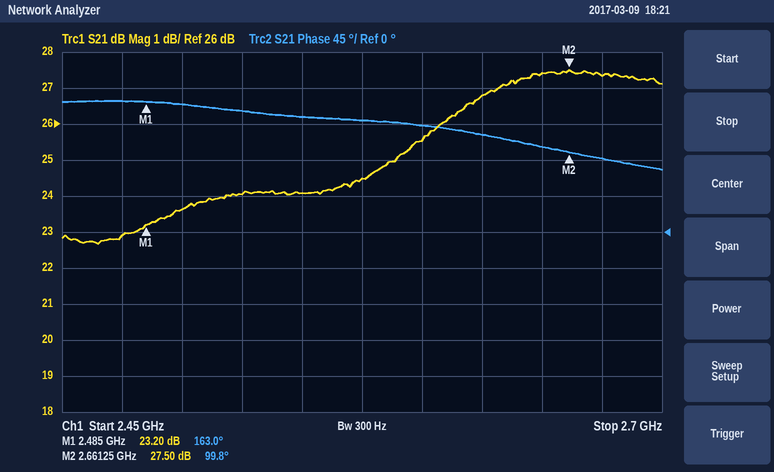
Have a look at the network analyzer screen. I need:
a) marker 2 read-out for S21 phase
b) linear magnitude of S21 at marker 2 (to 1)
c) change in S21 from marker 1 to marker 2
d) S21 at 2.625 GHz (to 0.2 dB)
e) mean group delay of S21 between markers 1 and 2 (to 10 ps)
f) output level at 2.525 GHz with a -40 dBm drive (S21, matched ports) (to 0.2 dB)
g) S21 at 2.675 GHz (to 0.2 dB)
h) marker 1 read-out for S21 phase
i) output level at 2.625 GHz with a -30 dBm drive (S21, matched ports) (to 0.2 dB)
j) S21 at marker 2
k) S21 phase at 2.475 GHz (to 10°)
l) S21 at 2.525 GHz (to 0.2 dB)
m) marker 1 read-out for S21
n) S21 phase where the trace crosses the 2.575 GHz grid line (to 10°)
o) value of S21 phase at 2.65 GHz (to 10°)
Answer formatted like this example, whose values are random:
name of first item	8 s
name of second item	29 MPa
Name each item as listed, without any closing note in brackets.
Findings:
marker 2 read-out for S21 phase	99.8°
linear magnitude of S21 at marker 2	24
change in S21 from marker 1 to marker 2	4.30 dB
S21 at 2.625 GHz	26.8 dB
mean group delay of S21 between markers 1 and 2	1.00 ns
output level at 2.525 GHz with a -40 dBm drive (S21, matched ports)	-16.0 dBm
S21 at 2.675 GHz	27.4 dB
marker 1 read-out for S21 phase	163.0°
output level at 2.625 GHz with a -30 dBm drive (S21, matched ports)	-3.2 dBm
S21 at marker 2	27.50 dB
S21 phase at 2.475 GHz	160°
S21 at 2.525 GHz	24.0 dB
marker 1 read-out for S21	23.20 dB
S21 phase where the trace crosses the 2.575 GHz grid line	140°
value of S21 phase at 2.65 GHz	110°
